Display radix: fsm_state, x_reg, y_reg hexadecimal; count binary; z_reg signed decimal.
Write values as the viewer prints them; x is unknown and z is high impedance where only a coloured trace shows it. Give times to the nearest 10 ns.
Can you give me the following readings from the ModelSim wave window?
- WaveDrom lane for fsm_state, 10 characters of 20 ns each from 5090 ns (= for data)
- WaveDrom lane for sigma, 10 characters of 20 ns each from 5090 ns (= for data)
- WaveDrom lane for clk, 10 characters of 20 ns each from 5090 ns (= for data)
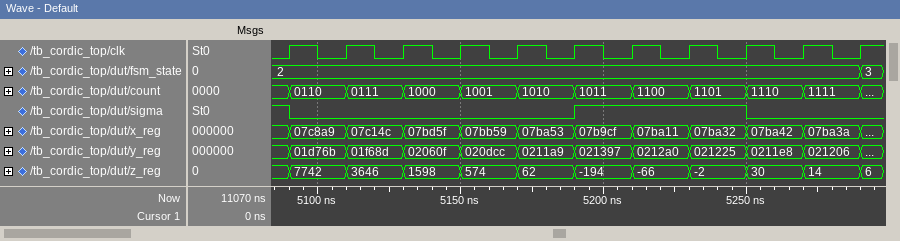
{name: 'fsm_state', wave: '=.........', data: '2'}
{name: 'sigma', wave: '0....1..0.'}
{name: 'clk', wave: 'p.........'}
